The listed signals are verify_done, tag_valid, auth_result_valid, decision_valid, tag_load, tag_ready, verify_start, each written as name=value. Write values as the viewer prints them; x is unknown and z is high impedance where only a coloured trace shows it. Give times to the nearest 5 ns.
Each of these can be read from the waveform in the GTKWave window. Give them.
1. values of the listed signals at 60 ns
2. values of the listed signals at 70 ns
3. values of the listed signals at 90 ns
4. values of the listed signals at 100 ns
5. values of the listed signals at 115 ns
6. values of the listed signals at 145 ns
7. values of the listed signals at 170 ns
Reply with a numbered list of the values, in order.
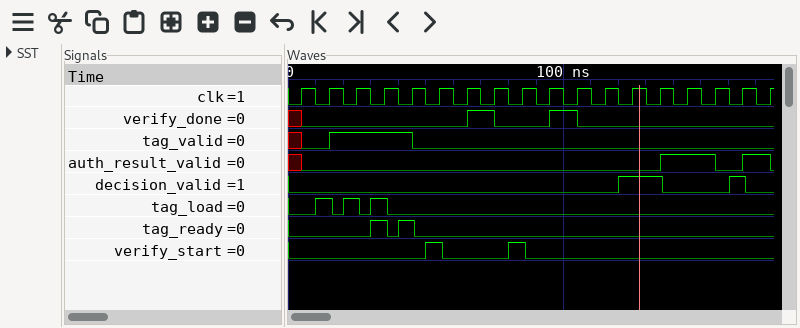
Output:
1. verify_done=0, tag_valid=0, auth_result_valid=0, decision_valid=0, tag_load=0, tag_ready=0, verify_start=0
2. verify_done=1, tag_valid=0, auth_result_valid=0, decision_valid=0, tag_load=0, tag_ready=0, verify_start=0
3. verify_done=0, tag_valid=0, auth_result_valid=0, decision_valid=0, tag_load=0, tag_ready=0, verify_start=0
4. verify_done=1, tag_valid=0, auth_result_valid=0, decision_valid=0, tag_load=0, tag_ready=0, verify_start=0
5. verify_done=0, tag_valid=0, auth_result_valid=0, decision_valid=0, tag_load=0, tag_ready=0, verify_start=0
6. verify_done=0, tag_valid=0, auth_result_valid=1, decision_valid=0, tag_load=0, tag_ready=0, verify_start=0
7. verify_done=0, tag_valid=0, auth_result_valid=1, decision_valid=0, tag_load=0, tag_ready=0, verify_start=0
